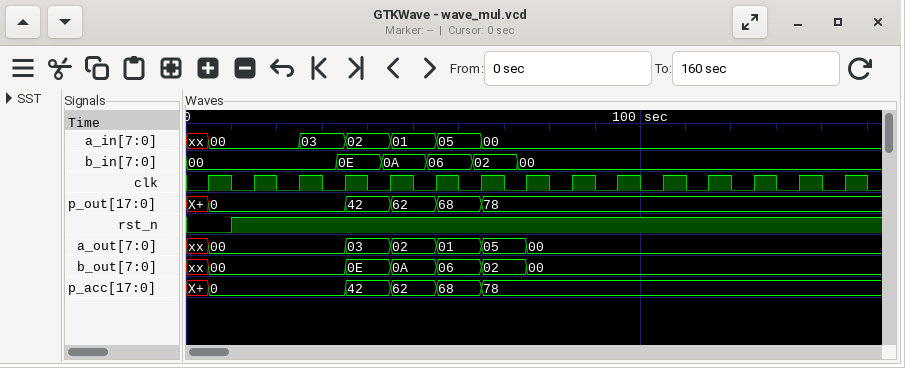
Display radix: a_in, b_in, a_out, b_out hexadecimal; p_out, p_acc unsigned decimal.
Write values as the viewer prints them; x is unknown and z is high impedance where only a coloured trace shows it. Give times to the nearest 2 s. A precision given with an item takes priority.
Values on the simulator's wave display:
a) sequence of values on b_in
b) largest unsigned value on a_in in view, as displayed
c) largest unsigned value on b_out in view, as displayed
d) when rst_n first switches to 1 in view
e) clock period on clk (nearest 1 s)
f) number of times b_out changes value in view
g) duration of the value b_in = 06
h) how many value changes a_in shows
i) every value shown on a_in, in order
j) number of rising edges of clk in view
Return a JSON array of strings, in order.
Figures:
["00, 0E, 0A, 06, 02, 00", "05", "0E", "10 s", "10 s", "6", "10 s", "6", "xx, 00, 03, 02, 01, 05, 00", "15"]
